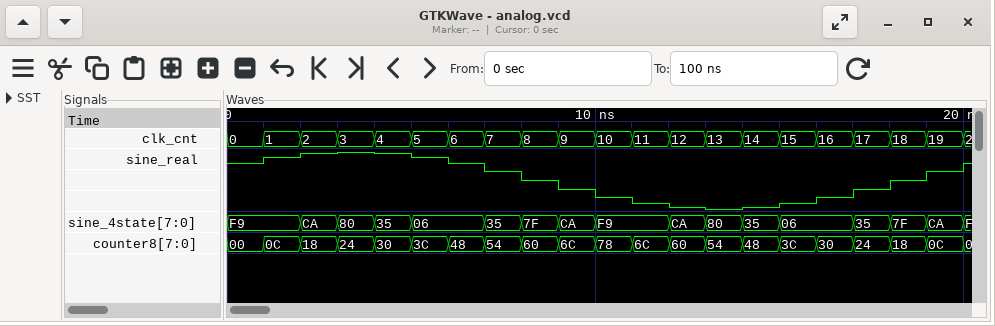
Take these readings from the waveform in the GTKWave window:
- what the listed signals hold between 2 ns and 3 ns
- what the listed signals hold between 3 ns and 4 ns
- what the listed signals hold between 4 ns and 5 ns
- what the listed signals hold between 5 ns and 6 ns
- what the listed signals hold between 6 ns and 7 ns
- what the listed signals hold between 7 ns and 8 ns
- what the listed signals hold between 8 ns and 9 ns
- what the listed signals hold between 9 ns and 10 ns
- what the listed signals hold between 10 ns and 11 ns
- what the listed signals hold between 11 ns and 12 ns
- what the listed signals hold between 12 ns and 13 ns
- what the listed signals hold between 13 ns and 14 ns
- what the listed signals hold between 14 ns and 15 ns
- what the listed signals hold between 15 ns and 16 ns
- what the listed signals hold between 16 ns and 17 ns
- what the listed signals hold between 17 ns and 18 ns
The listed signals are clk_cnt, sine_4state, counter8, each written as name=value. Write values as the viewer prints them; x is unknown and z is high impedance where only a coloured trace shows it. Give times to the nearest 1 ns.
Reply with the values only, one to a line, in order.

clk_cnt=2, sine_4state=CA, counter8=18
clk_cnt=3, sine_4state=80, counter8=24
clk_cnt=4, sine_4state=35, counter8=30
clk_cnt=5, sine_4state=06, counter8=3C
clk_cnt=6, sine_4state=06, counter8=48
clk_cnt=7, sine_4state=35, counter8=54
clk_cnt=8, sine_4state=7F, counter8=60
clk_cnt=9, sine_4state=CA, counter8=6C
clk_cnt=10, sine_4state=F9, counter8=78
clk_cnt=11, sine_4state=F9, counter8=6C
clk_cnt=12, sine_4state=CA, counter8=60
clk_cnt=13, sine_4state=80, counter8=54
clk_cnt=14, sine_4state=35, counter8=48
clk_cnt=15, sine_4state=06, counter8=3C
clk_cnt=16, sine_4state=06, counter8=30
clk_cnt=17, sine_4state=35, counter8=24
